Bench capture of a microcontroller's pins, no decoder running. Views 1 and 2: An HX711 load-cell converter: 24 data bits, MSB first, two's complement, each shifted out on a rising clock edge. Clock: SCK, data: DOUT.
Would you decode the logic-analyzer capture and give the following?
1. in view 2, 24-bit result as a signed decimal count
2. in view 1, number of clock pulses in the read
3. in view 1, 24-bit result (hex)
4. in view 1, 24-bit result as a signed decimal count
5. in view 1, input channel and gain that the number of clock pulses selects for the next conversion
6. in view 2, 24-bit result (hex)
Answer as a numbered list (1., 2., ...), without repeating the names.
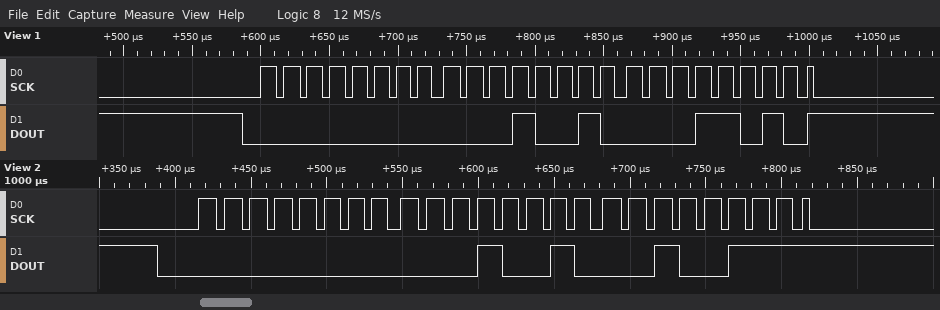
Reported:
1. 4647
2. 25
3. 0x00121A
4. 4634
5. channel A, gain 128
6. 0x001227
